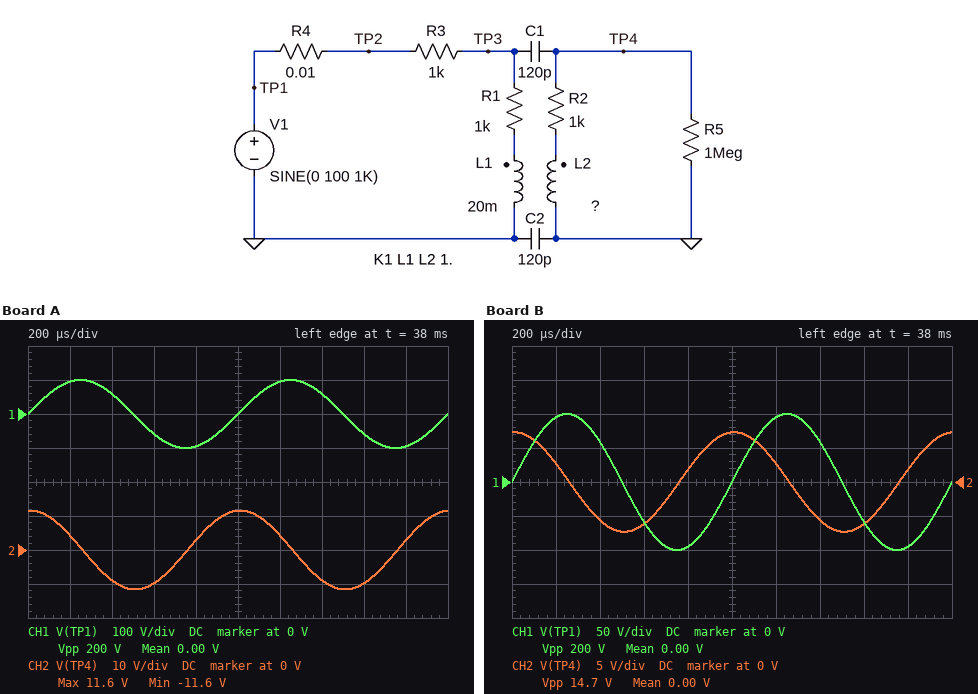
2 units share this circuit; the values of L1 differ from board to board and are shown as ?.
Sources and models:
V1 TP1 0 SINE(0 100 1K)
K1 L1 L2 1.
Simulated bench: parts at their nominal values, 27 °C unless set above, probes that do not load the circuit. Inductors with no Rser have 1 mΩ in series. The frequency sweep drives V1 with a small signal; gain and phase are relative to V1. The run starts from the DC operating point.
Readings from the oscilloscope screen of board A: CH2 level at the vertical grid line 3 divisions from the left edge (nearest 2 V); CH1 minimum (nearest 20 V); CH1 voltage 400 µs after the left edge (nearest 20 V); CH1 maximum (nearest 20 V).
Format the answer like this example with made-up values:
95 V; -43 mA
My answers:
-10 V; -100 V; 60 V; 100 V
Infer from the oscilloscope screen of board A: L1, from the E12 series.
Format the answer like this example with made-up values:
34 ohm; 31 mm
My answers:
68 mH
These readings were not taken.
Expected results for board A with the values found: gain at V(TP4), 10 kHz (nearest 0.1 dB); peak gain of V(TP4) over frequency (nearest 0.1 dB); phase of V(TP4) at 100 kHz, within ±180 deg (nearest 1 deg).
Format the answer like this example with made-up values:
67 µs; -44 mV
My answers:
-0.1 dB; 5.2 dB; -2 deg
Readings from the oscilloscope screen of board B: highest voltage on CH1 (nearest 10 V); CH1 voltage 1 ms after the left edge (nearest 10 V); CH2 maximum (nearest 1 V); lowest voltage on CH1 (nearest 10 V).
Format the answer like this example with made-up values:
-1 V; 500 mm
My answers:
100 V; 0 V; 7 V; -100 V
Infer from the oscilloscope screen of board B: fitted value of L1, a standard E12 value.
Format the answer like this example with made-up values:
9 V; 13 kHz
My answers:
27 mH
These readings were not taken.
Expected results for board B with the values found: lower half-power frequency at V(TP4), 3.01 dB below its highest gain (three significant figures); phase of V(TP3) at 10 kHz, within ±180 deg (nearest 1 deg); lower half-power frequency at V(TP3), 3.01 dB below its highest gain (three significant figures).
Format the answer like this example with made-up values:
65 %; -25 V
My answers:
15.6 kHz; 19 deg; 11.2 kHz
